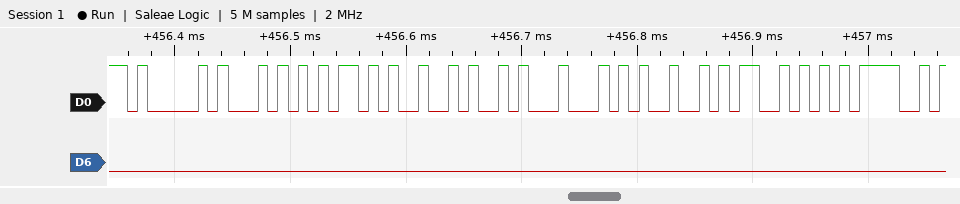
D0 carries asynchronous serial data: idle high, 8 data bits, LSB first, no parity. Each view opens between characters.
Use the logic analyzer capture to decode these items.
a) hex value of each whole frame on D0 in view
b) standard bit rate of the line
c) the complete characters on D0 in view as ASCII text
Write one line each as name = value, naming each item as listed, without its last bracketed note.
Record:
hex value of each whole frame on D0 in view = 41, 54, 2B, 4A, 44, 49, 53, 3D
standard bit rate of the line = 115200 baud
the complete characters on D0 in view as ASCII text = "AT+JDIS="
